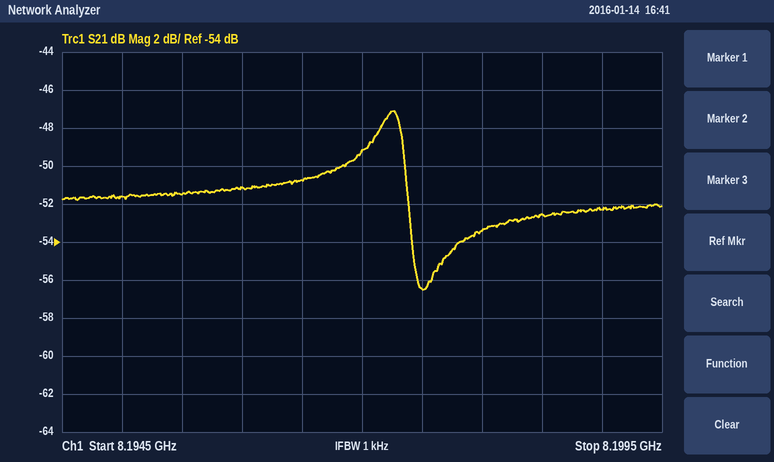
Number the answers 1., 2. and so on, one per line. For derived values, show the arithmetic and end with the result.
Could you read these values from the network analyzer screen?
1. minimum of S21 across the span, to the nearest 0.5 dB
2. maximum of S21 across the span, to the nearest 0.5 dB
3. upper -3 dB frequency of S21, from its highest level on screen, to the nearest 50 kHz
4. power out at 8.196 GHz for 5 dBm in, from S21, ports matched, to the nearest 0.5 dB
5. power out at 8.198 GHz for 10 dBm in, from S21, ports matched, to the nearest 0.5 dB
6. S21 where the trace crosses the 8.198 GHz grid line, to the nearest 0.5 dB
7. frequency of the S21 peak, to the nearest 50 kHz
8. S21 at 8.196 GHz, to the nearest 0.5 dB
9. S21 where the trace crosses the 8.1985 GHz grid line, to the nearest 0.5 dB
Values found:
1. -56.5 dB
2. -47.0 dB
3. 8.19735 GHz
4. 5 dBm + (-51.0 dB) = -46.0 dBm
5. 10 dBm + (-53.5 dB) = -43.5 dBm
6. -53.5 dB
7. 8.19725 GHz
8. -51.0 dB
9. -52.5 dB
